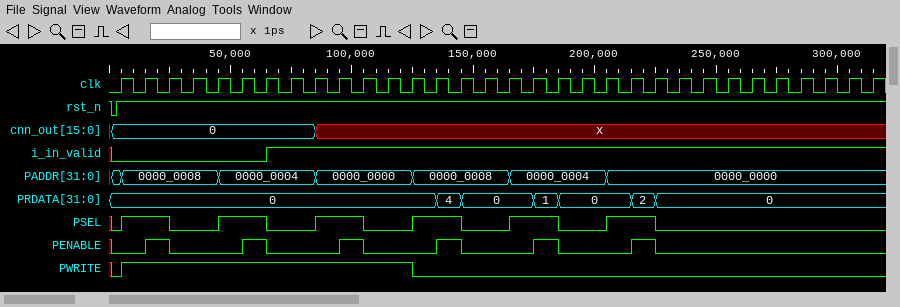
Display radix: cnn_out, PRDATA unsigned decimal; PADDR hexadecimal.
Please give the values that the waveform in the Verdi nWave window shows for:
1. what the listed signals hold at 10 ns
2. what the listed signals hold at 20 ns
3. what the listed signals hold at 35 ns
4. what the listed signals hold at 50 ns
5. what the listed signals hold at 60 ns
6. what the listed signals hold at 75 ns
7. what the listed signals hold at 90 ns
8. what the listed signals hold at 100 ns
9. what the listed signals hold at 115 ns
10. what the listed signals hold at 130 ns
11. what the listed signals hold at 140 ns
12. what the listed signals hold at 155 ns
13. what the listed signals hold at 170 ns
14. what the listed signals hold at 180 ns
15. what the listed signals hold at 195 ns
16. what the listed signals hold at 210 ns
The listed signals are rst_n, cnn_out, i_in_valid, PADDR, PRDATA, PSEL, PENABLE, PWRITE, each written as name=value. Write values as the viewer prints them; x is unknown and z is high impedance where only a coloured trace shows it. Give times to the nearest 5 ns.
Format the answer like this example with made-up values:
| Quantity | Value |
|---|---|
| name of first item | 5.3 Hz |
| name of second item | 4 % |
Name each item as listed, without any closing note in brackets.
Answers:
| Quantity | Value |
|---|---|
| what the listed signals hold at 10 ns | rst_n=1, cnn_out=0, i_in_valid=0, PADDR=0000_0008, PRDATA=0, PSEL=1, PENABLE=0, PWRITE=1 |
| what the listed signals hold at 20 ns | rst_n=1, cnn_out=0, i_in_valid=0, PADDR=0000_0008, PRDATA=0, PSEL=1, PENABLE=1, PWRITE=1 |
| what the listed signals hold at 35 ns | rst_n=1, cnn_out=0, i_in_valid=0, PADDR=0000_0008, PRDATA=0, PSEL=0, PENABLE=0, PWRITE=1 |
| what the listed signals hold at 50 ns | rst_n=1, cnn_out=0, i_in_valid=0, PADDR=0000_0004, PRDATA=0, PSEL=1, PENABLE=0, PWRITE=1 |
| what the listed signals hold at 60 ns | rst_n=1, cnn_out=0, i_in_valid=0, PADDR=0000_0004, PRDATA=0, PSEL=1, PENABLE=1, PWRITE=1 |
| what the listed signals hold at 75 ns | rst_n=1, cnn_out=0, i_in_valid=1, PADDR=0000_0004, PRDATA=0, PSEL=0, PENABLE=0, PWRITE=1 |
| what the listed signals hold at 90 ns | rst_n=1, cnn_out=x, i_in_valid=1, PADDR=0000_0000, PRDATA=0, PSEL=1, PENABLE=0, PWRITE=1 |
| what the listed signals hold at 100 ns | rst_n=1, cnn_out=x, i_in_valid=1, PADDR=0000_0000, PRDATA=0, PSEL=1, PENABLE=1, PWRITE=1 |
| what the listed signals hold at 115 ns | rst_n=1, cnn_out=x, i_in_valid=1, PADDR=0000_0000, PRDATA=0, PSEL=0, PENABLE=0, PWRITE=1 |
| what the listed signals hold at 130 ns | rst_n=1, cnn_out=x, i_in_valid=1, PADDR=0000_0008, PRDATA=0, PSEL=1, PENABLE=0, PWRITE=0 |
| what the listed signals hold at 140 ns | rst_n=1, cnn_out=x, i_in_valid=1, PADDR=0000_0008, PRDATA=4, PSEL=1, PENABLE=1, PWRITE=0 |
| what the listed signals hold at 155 ns | rst_n=1, cnn_out=x, i_in_valid=1, PADDR=0000_0008, PRDATA=0, PSEL=0, PENABLE=0, PWRITE=0 |
| what the listed signals hold at 170 ns | rst_n=1, cnn_out=x, i_in_valid=1, PADDR=0000_0004, PRDATA=0, PSEL=1, PENABLE=0, PWRITE=0 |
| what the listed signals hold at 180 ns | rst_n=1, cnn_out=x, i_in_valid=1, PADDR=0000_0004, PRDATA=1, PSEL=1, PENABLE=1, PWRITE=0 |
| what the listed signals hold at 195 ns | rst_n=1, cnn_out=x, i_in_valid=1, PADDR=0000_0004, PRDATA=0, PSEL=0, PENABLE=0, PWRITE=0 |
| what the listed signals hold at 210 ns | rst_n=1, cnn_out=x, i_in_valid=1, PADDR=0000_0000, PRDATA=0, PSEL=1, PENABLE=0, PWRITE=0 |
